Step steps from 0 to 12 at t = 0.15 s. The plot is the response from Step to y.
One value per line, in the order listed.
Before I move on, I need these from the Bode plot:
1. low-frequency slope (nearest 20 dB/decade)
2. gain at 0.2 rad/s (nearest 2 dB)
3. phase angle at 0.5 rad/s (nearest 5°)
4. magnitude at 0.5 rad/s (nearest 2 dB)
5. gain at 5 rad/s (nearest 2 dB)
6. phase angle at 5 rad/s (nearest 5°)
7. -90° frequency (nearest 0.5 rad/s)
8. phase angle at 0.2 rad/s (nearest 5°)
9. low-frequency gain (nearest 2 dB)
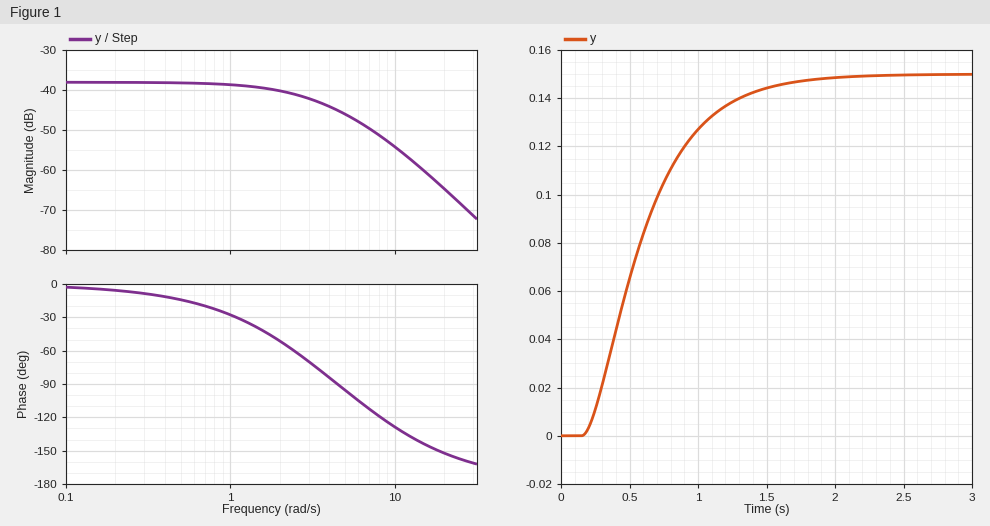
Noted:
0 dB/decade
-38 dB
-15°
-38 dB
-46 dB
-95°
4.5 rad/s
-5°
-38 dB
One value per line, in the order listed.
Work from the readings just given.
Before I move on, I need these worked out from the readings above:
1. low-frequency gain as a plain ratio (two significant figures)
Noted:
0.013
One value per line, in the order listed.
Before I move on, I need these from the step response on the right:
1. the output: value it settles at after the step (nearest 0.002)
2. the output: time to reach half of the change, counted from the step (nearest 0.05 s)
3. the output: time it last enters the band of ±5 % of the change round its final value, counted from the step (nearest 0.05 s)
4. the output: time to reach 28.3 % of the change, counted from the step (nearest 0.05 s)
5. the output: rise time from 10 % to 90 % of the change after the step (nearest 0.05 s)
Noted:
0.150
0.40 s
1.25 s
0.25 s
0.90 s
